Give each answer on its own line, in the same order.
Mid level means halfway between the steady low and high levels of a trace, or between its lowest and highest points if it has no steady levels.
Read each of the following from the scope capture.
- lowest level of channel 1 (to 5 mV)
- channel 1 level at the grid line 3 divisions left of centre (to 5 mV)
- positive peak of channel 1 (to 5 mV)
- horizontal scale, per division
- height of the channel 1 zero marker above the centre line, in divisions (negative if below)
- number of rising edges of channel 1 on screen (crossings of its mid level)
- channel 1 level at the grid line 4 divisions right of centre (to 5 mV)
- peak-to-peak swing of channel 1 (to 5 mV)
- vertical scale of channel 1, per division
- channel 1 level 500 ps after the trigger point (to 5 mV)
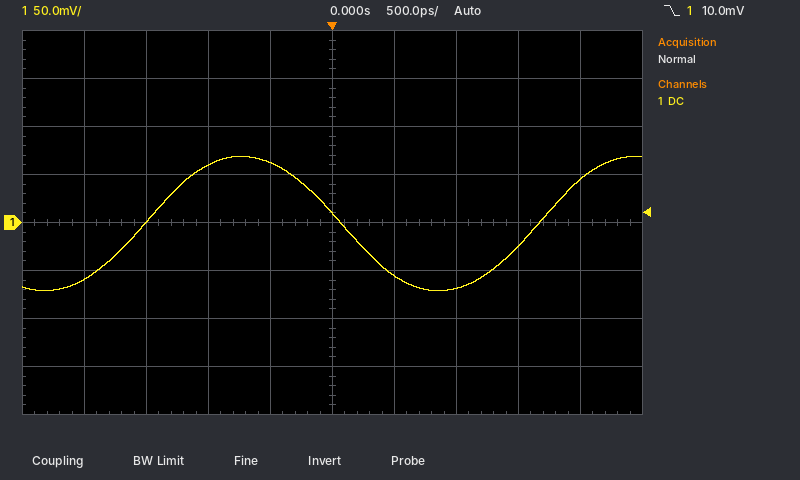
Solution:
-70 mV
0 mV
70 mV
500 ps
0.0 div
2
45 mV
140 mV
50 mV
-55 mV
